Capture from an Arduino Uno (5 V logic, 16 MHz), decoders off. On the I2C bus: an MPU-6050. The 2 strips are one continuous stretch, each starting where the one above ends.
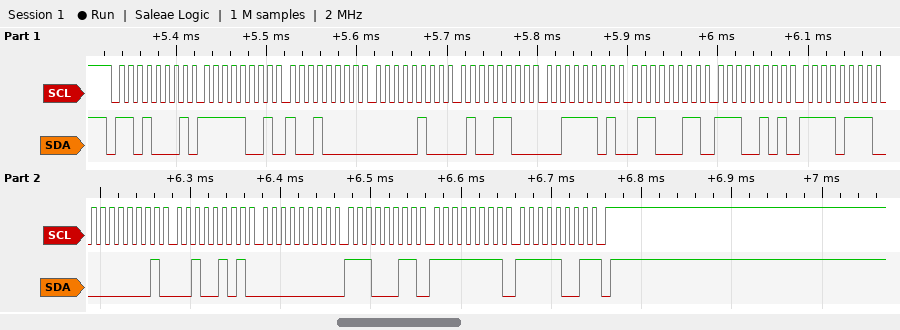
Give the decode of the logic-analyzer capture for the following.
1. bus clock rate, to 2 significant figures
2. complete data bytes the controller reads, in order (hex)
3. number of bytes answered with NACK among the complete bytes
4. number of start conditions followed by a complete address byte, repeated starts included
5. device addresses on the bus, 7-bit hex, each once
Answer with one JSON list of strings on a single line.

["100 kHz", "F9 90 04 4C 3D 63 E5 F7 01 25 00 E3 FF F9", "1", "1", "0x68"]
